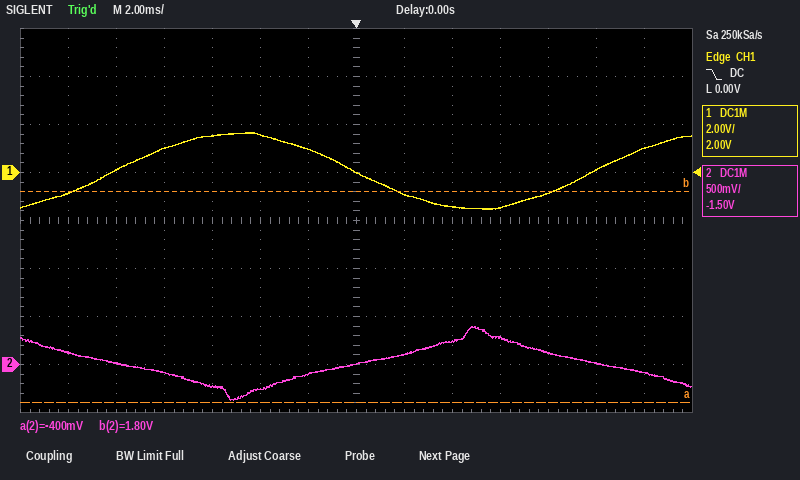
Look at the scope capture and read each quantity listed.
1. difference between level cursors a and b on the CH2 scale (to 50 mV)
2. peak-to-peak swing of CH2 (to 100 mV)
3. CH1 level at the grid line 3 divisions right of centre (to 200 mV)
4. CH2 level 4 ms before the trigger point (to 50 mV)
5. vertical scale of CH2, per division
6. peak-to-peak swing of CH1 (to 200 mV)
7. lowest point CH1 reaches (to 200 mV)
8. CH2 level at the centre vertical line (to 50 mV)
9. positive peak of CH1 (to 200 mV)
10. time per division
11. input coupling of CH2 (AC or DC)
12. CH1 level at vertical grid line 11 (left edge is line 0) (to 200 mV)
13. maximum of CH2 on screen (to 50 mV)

2.20 V
800 mV
-1.4 V
-250 mV
500 mV
3.2 V
-1.6 V
0 mV
1.6 V
2 ms
DC
-800 mV
400 mV
